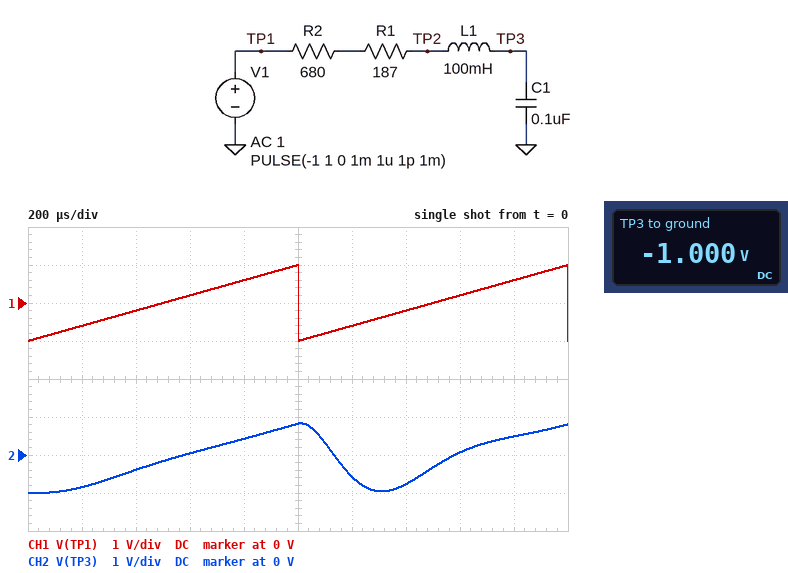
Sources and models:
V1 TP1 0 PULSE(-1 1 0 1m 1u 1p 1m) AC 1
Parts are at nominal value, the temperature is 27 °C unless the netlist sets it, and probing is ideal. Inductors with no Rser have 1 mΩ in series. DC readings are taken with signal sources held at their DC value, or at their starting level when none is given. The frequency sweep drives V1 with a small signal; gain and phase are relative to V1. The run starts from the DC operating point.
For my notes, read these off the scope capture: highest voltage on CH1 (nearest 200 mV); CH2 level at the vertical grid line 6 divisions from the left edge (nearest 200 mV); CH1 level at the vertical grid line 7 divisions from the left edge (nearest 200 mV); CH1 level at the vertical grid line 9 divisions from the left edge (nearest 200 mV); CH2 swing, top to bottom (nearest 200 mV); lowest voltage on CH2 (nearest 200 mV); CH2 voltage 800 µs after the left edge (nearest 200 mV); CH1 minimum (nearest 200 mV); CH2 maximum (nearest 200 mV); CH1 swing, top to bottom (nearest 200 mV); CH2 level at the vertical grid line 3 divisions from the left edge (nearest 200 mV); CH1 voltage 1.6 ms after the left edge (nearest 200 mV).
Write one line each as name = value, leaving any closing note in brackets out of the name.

highest voltage on CH1 = 1.0 V
CH2 level at the vertical grid line 6 divisions from the left edge = -600 mV
CH1 level at the vertical grid line 7 divisions from the left edge = -200 mV
CH1 level at the vertical grid line 9 divisions from the left edge = 600 mV
CH2 swing, top to bottom = 1.8 V
lowest voltage on CH2 = -1.0 V
CH2 voltage 800 µs after the left edge = 400 mV
CH1 minimum = -1.0 V
CH2 maximum = 800 mV
CH1 swing, top to bottom = 2.0 V
CH2 level at the vertical grid line 3 divisions from the left edge = 0 V
CH1 voltage 1.6 ms after the left edge = 200 mV
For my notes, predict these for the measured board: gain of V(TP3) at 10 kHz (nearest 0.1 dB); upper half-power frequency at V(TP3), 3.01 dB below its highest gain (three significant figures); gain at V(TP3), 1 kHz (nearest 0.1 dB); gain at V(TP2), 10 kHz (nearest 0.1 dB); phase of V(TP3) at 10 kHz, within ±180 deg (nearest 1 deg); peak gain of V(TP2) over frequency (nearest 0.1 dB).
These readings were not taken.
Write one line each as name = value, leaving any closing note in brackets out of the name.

gain of V(TP3) at 10 kHz = -31.8 dB
upper half-power frequency at V(TP3), 3.01 dB below its highest gain = 1.89 kHz
gain at V(TP3), 1 kHz = 1.8 dB
gain at V(TP2), 10 kHz = -0.1 dB
phase of V(TP3) at 10 kHz, within ±180 deg = -172 deg
peak gain of V(TP2) over frequency = 0 dB
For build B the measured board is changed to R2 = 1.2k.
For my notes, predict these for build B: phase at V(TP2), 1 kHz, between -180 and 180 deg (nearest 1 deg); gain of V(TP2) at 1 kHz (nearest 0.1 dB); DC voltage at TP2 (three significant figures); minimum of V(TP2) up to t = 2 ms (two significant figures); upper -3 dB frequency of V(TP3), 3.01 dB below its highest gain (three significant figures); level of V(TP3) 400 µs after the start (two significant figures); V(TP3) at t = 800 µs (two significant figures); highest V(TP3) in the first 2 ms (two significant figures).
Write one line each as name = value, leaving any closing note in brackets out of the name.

phase at V(TP2), 1 kHz, between -180 and 180 deg = -55 deg
gain of V(TP2) at 1 kHz = -4.9 dB
DC voltage at TP2 = -1.00 V
minimum of V(TP2) up to t = 2 ms = -1.3 V
upper -3 dB frequency of V(TP3), 3.01 dB below its highest gain = 1.62 kHz
level of V(TP3) 400 µs after the start = -490 mV
V(TP3) at t = 800 µs = 320 mV
highest V(TP3) in the first 2 ms = 730 mV
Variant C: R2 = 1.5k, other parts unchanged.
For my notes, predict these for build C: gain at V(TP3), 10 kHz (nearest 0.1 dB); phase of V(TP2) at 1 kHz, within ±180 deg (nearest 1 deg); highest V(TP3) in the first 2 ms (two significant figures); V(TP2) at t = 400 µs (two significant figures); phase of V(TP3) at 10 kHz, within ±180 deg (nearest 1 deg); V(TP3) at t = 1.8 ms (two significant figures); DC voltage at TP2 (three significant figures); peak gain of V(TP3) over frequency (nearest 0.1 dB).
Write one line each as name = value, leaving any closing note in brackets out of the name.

gain at V(TP3), 10 kHz = -32.0 dB
phase of V(TP2) at 1 kHz, within ±180 deg = -60 deg
highest V(TP3) in the first 2 ms = 670 mV
V(TP2) at t = 400 µs = -530 mV
phase of V(TP3) at 10 kHz, within ±180 deg = -165 deg
V(TP3) at t = 1.8 ms = 260 mV
DC voltage at TP2 = -1.00 V
peak gain of V(TP3) over frequency = 0 dB
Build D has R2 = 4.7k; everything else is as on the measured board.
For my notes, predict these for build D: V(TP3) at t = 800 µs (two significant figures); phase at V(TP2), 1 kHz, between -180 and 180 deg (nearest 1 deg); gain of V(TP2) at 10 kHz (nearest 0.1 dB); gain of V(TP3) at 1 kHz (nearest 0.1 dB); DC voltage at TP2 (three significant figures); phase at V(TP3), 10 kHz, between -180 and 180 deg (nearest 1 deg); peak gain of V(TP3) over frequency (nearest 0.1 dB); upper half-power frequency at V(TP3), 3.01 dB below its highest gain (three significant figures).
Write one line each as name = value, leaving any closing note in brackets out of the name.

V(TP3) at t = 800 µs = -200 mV
phase at V(TP2), 1 kHz, between -180 and 180 deg = -79 deg
gain of V(TP2) at 10 kHz = -2.1 dB
gain of V(TP3) at 1 kHz = -9.9 dB
DC voltage at TP2 = -1.00 V
phase at V(TP3), 10 kHz, between -180 and 180 deg = -141 deg
peak gain of V(TP3) over frequency = 0 dB
upper half-power frequency at V(TP3), 3.01 dB below its highest gain = 340 Hz
